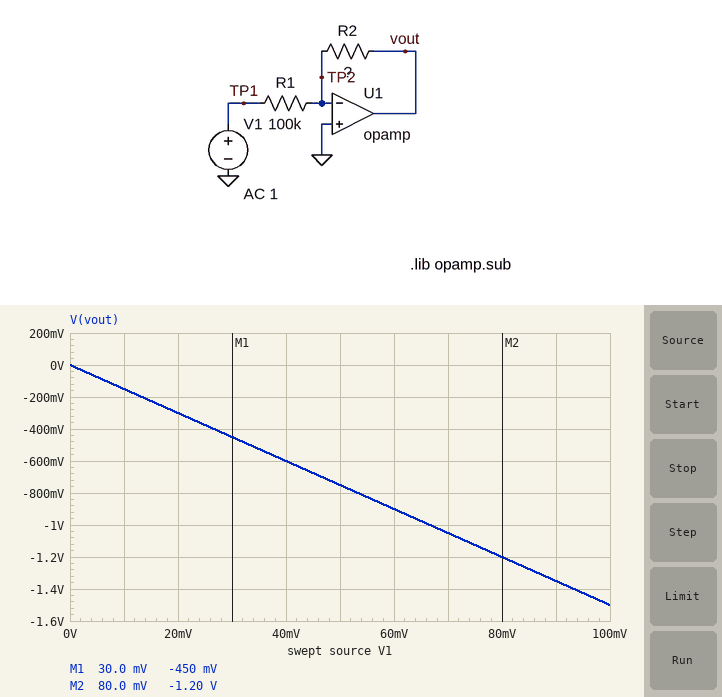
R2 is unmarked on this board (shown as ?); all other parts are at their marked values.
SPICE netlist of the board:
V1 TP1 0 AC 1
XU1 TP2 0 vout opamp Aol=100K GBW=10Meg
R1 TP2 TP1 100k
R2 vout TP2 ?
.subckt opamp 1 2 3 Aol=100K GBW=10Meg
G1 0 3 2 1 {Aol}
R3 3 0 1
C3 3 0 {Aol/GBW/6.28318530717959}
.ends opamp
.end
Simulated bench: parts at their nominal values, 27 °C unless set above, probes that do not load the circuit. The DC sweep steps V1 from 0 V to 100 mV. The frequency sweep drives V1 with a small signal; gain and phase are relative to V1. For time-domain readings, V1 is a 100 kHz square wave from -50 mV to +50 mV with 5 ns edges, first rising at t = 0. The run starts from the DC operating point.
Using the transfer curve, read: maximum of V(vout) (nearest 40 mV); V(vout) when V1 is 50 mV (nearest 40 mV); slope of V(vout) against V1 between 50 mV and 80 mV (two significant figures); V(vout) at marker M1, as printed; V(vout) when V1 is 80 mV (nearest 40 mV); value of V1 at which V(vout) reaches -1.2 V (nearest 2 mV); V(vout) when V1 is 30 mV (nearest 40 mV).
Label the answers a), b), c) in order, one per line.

a) 0 V
b) -760 mV
c) -15 V/V
d) -450 mV
e) -1.20 V
f) 80 mV
g) -440 mV
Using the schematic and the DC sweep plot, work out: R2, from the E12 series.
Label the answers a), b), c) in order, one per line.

a) 1.5 MΩ
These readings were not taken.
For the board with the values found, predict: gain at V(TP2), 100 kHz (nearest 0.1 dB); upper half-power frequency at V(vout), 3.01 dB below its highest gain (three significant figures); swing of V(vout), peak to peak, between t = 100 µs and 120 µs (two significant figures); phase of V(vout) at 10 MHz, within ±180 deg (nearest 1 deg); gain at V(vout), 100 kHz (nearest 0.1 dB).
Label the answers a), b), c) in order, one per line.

a) -16.6 dB
b) 625 kHz
c) 1.5 V
d) 94 deg
e) 23.4 dB
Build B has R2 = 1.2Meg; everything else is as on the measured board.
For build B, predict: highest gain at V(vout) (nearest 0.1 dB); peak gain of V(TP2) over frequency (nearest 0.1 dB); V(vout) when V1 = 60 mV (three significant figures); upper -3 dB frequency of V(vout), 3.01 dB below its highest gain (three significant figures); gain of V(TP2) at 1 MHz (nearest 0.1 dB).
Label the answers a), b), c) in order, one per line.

a) 21.6 dB
b) -0.7 dB
c) -720 mV
d) 769 kHz
e) -2.7 dB
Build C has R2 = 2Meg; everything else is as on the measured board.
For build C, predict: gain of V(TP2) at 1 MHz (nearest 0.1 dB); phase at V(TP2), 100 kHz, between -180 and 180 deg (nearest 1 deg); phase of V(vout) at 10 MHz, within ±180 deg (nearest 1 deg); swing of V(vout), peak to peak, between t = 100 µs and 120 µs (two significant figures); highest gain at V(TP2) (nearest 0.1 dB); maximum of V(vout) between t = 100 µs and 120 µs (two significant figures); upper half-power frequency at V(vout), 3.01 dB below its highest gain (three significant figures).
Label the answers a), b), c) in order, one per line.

a) -1.3 dB
b) 78 deg
c) 93 deg
d) 2.0 V
e) -0.4 dB
f) 1.0 V
g) 476 kHz
